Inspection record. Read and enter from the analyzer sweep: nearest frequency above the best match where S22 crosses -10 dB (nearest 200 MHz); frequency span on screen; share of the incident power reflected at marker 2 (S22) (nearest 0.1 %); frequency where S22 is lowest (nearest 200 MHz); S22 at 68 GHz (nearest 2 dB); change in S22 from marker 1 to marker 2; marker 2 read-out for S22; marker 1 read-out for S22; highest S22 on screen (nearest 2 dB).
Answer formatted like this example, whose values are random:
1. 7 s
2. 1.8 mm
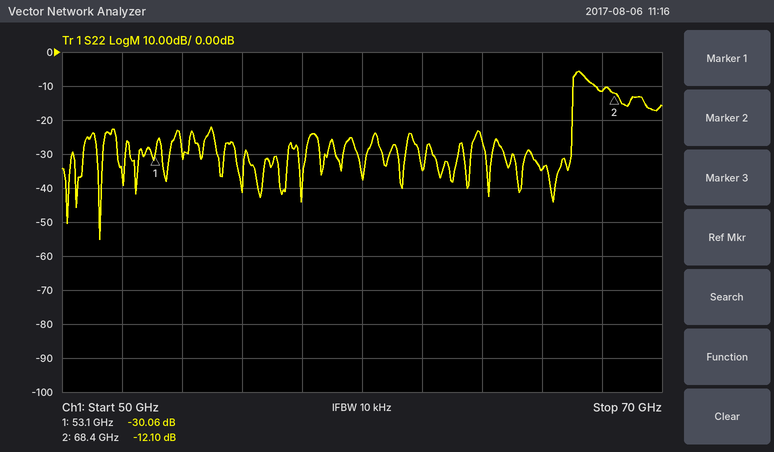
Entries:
1. 67.0 GHz
2. 20 GHz
3. 6.2 %
4. 51.2 GHz
5. -12 dB
6. 17.96 dB
7. -12.10 dB
8. -30.06 dB
9. -6 dB
